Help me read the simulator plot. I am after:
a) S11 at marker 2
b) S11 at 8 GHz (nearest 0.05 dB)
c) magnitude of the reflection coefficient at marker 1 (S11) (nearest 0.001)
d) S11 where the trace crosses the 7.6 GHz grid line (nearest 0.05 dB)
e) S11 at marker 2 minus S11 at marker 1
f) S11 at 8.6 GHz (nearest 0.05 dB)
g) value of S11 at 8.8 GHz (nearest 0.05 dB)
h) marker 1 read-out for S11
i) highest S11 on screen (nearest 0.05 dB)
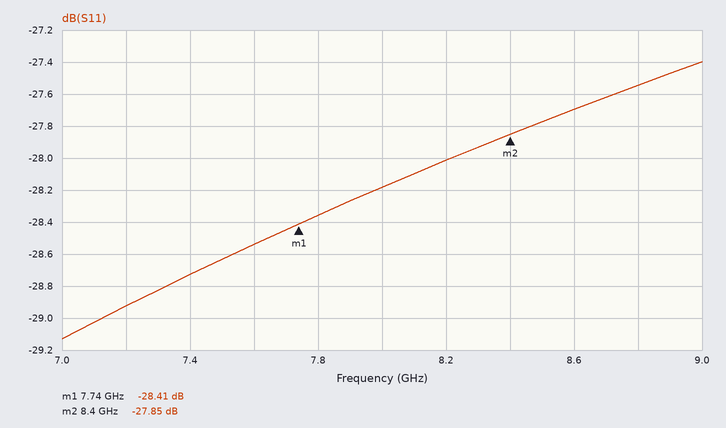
-27.85 dB
-28.20 dB
0.038
-28.55 dB
0.56 dB
-27.70 dB
-27.55 dB
-28.41 dB
-27.40 dB
